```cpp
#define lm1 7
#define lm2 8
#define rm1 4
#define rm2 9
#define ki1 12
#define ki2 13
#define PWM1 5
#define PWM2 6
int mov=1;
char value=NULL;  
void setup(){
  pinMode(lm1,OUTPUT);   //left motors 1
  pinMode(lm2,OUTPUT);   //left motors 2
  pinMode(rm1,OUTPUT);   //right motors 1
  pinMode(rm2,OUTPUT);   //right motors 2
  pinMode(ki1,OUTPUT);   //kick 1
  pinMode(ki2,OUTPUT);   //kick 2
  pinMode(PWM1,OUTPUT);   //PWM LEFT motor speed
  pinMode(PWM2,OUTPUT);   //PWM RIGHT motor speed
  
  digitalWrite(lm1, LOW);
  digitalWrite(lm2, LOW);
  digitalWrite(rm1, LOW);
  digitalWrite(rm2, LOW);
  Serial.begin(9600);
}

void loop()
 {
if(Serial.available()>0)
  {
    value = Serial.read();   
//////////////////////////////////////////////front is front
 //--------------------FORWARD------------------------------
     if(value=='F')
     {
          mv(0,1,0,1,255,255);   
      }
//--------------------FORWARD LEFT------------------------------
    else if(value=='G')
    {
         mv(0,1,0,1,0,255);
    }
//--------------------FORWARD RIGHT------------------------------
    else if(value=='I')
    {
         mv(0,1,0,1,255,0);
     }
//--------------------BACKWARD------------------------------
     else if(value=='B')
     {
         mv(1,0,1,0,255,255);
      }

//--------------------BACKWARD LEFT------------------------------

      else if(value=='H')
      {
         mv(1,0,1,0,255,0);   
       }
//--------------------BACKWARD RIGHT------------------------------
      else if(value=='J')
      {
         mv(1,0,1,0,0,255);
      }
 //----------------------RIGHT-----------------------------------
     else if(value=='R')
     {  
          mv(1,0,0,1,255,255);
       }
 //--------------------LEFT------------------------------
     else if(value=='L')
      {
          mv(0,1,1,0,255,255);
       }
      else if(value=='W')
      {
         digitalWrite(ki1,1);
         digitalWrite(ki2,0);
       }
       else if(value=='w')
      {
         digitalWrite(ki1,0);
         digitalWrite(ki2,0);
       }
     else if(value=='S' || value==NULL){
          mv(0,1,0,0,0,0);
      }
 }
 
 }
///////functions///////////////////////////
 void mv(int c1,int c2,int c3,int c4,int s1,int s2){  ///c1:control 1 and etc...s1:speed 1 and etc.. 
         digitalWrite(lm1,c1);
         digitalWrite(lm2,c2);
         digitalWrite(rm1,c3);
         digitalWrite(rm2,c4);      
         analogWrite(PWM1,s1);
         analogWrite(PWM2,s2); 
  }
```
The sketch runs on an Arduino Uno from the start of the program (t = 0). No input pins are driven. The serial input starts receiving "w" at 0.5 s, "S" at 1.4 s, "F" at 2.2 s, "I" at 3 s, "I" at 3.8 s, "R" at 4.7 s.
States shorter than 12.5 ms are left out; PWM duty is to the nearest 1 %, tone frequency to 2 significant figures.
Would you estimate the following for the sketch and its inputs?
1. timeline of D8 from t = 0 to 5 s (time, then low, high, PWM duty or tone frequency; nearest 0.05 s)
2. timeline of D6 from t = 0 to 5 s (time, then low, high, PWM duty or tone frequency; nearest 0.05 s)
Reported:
0 s low; 1.4 s high; 4.7 s low
0 s low; 2.2 s high; 3 s low; 4.7 s high
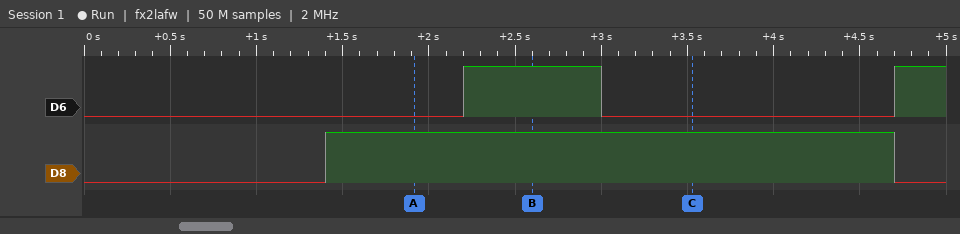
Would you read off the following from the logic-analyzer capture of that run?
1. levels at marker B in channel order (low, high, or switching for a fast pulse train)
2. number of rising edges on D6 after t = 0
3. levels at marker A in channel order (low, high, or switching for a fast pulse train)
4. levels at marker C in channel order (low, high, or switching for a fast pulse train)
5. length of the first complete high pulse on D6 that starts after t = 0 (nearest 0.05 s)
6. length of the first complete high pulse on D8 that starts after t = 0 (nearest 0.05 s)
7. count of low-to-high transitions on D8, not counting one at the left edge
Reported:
D6 high, D8 high
2
D6 low, D8 high
D6 low, D8 high
0.80 s
3.30 s
1
